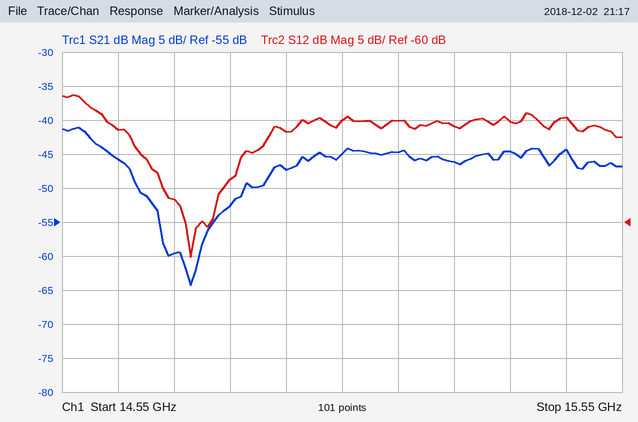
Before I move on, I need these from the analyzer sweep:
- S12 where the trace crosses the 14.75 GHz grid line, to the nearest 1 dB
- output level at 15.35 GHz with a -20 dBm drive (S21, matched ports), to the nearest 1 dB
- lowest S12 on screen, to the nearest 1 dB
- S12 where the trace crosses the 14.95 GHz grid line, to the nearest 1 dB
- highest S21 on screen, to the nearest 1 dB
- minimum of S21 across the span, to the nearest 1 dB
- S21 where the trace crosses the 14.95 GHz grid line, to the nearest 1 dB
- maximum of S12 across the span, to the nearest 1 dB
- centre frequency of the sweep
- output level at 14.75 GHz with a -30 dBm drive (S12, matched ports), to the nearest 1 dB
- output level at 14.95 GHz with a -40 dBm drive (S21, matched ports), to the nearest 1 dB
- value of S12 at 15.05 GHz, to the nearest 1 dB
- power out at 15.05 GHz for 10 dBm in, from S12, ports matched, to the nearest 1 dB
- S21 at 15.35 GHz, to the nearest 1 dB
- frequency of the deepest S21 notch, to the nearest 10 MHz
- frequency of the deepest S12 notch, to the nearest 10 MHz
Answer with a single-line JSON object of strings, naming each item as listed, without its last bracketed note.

{"S12 where the trace crosses the 14.75 GHz grid line, to the nearest 1 dB": "-57 dB", "output level at 15.35 GHz with a -20 dBm drive (S21, matched ports), to the nearest 1 dB": "-65 dBm", "lowest S12 on screen, to the nearest 1 dB": "-65 dB", "S12 where the trace crosses the 14.95 GHz grid line, to the nearest 1 dB": "-47 dB", "highest S21 on screen, to the nearest 1 dB": "-41 dB", "minimum of S21 across the span, to the nearest 1 dB": "-64 dB", "S21 where the trace crosses the 14.95 GHz grid line, to the nearest 1 dB": "-47 dB", "maximum of S12 across the span, to the nearest 1 dB": "-41 dB", "centre frequency of the sweep": "15.05 GHz", "output level at 14.75 GHz with a -30 dBm drive (S12, matched ports), to the nearest 1 dB": "-87 dBm", "output level at 14.95 GHz with a -40 dBm drive (S21, matched ports), to the nearest 1 dB": "-87 dBm", "value of S12 at 15.05 GHz, to the nearest 1 dB": "-45 dB", "power out at 15.05 GHz for 10 dBm in, from S12, ports matched, to the nearest 1 dB": "-35 dBm", "S21 at 15.35 GHz, to the nearest 1 dB": "-45 dB", "frequency of the deepest S21 notch, to the nearest 10 MHz": "14.78 GHz", "frequency of the deepest S12 notch, to the nearest 10 MHz": "14.78 GHz"}
